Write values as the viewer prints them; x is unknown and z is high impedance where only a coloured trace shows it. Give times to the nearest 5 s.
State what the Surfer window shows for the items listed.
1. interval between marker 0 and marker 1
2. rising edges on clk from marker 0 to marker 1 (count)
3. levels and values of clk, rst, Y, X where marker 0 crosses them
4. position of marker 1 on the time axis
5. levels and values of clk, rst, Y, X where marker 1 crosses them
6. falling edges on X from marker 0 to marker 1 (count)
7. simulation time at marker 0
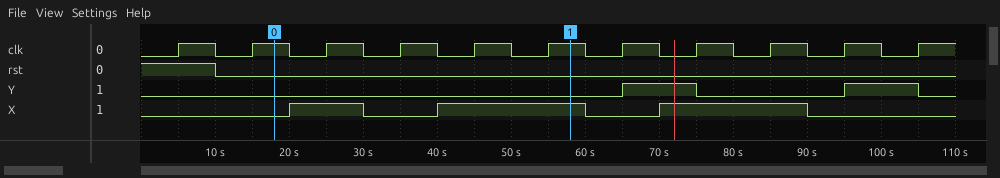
40 s
4
clk=1, rst=0, Y=0, X=0
60 s
clk=1, rst=0, Y=0, X=1
1
20 s
